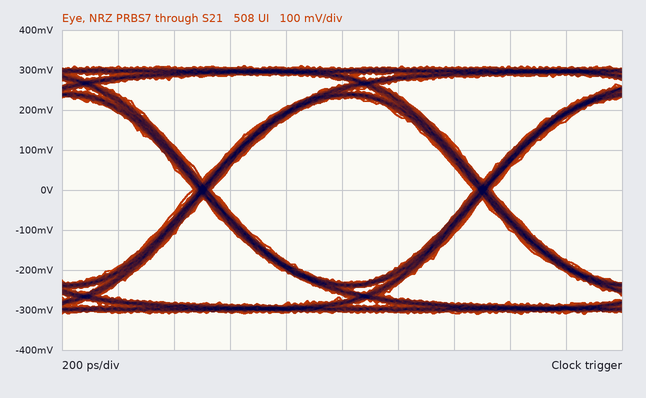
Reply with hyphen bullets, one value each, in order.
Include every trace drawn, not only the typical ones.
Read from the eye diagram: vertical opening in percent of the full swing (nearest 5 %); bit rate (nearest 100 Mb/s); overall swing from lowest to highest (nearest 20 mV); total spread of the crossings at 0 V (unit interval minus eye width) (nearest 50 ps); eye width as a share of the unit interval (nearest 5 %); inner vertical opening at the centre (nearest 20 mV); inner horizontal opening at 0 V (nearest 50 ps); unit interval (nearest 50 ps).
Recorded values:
- 75 %
- 1.0 Gb/s
- 620 mV
- 50 ps
- 95 %
- 460 mV
- 950 ps
- 1.00 ns
